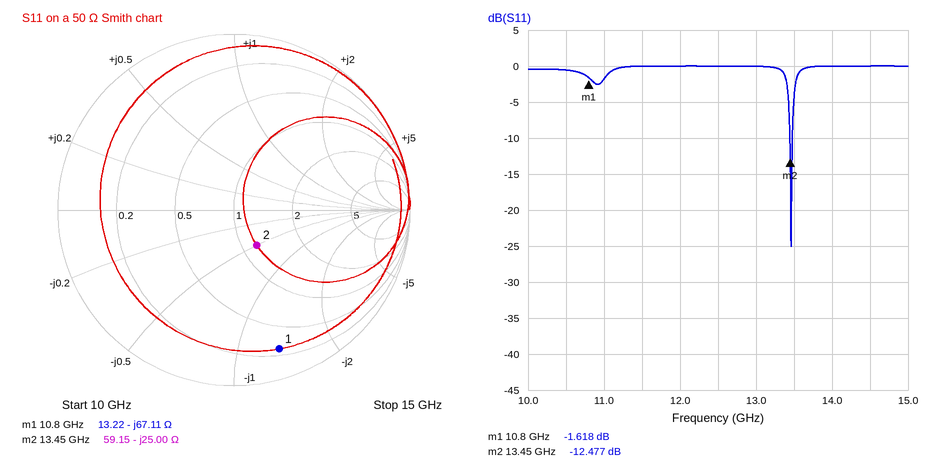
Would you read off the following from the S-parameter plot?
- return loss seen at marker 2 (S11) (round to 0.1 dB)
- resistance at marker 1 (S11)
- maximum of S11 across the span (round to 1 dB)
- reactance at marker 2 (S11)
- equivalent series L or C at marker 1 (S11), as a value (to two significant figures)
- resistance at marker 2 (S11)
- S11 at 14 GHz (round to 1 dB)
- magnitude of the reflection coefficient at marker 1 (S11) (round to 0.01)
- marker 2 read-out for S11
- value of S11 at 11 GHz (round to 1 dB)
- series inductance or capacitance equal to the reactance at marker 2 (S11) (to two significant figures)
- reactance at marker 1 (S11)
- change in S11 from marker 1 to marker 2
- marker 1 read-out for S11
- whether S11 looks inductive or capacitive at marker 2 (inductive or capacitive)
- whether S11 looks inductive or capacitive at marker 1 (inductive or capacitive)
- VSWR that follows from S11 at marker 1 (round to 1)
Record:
12.5 dB
13.22 Ω
0 dB
-25.00 Ω
220 fF
59.15 Ω
0 dB
0.83
-12.477 dB
-2 dB
470 fF
-67.11 Ω
-10.859 dB
-1.618 dB
capacitive
capacitive
11
